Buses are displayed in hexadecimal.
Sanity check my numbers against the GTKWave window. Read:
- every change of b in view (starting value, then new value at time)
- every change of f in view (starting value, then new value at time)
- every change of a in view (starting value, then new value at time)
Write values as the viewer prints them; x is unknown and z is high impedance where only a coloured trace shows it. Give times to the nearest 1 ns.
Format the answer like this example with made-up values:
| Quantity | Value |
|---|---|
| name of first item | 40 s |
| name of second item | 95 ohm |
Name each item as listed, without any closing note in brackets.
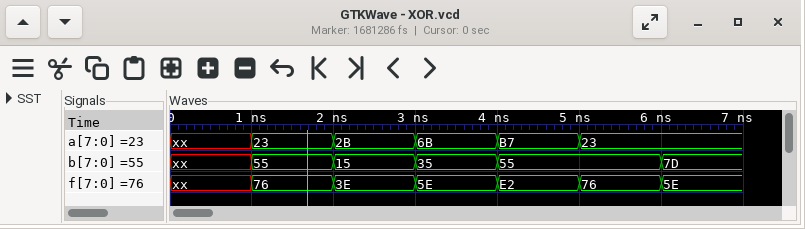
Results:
| Quantity | Value |
|---|---|
| every change of b in view | xx, 55 at 1 ns, 15 at 2 ns, 35 at 3 ns, 55 at 4 ns, 7D at 6 ns |
| every change of f in view | xx, 76 at 1 ns, 3E at 2 ns, 5E at 3 ns, E2 at 4 ns, 76 at 5 ns, 5E at 6 ns |
| every change of a in view | xx, 23 at 1 ns, 2B at 2 ns, 6B at 3 ns, B7 at 4 ns, 23 at 5 ns |
